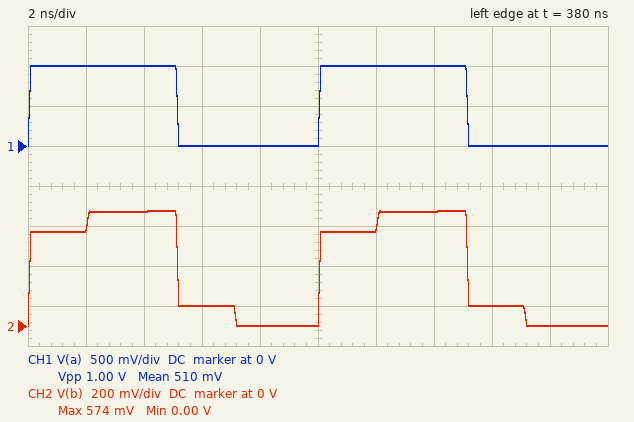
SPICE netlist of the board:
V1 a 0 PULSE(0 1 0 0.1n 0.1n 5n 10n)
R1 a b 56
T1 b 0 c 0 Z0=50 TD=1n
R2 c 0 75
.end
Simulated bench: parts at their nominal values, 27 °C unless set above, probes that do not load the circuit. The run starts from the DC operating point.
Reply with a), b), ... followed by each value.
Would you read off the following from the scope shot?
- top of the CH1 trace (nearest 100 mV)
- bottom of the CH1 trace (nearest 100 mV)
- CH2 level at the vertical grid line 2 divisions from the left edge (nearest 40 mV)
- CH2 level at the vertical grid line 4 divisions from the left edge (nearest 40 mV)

a) 1.0 V
b) 0 V
c) 560 mV
d) 0 V
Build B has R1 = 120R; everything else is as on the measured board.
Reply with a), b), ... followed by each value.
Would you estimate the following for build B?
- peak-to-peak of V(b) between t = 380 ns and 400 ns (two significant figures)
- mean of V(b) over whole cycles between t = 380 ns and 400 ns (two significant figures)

a) 380 mV
b) 200 mV
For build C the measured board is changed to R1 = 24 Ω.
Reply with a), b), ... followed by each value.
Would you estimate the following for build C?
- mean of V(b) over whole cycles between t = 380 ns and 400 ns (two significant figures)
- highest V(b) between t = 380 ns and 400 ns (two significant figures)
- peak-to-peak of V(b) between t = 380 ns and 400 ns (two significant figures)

a) 390 mV
b) 760 mV
c) 770 mV
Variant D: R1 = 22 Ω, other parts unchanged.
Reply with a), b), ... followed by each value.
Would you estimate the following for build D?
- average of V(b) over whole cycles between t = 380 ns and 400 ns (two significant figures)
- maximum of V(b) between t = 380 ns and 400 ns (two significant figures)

a) 390 mV
b) 780 mV
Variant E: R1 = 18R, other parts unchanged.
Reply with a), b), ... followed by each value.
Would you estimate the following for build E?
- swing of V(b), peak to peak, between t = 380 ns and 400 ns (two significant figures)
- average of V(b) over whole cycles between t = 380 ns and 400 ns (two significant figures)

a) 820 mV
b) 410 mV
